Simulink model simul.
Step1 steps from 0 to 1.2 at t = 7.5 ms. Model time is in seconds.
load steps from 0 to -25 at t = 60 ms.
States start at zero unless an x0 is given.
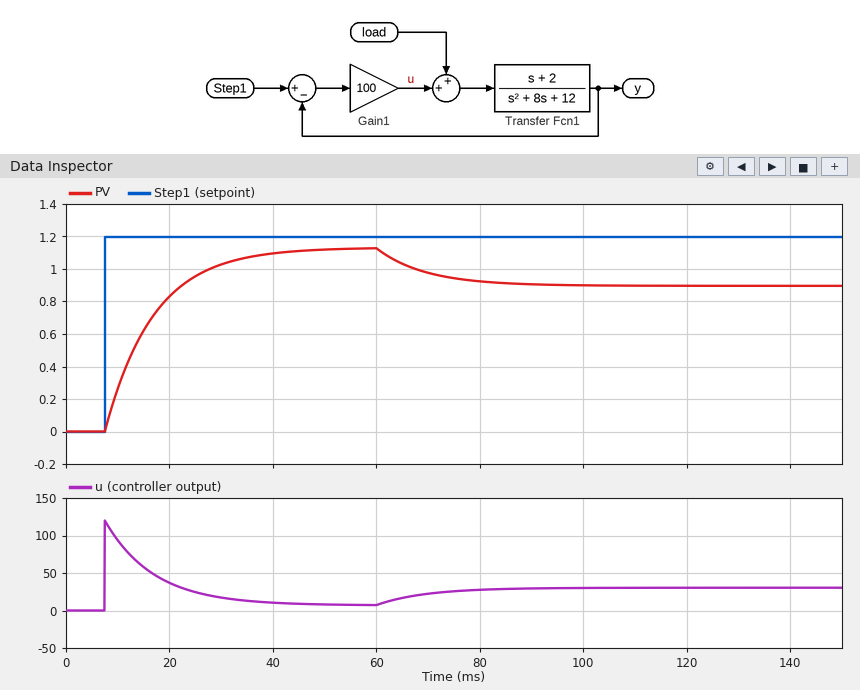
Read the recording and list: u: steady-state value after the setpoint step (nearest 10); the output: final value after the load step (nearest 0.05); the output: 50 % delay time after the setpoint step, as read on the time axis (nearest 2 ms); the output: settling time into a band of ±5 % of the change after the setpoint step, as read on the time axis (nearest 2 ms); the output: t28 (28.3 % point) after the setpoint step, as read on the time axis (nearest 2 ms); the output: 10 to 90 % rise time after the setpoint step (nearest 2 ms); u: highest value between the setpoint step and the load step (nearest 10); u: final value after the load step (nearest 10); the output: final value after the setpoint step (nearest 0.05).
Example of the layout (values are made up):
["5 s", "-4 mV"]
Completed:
["10", "0.90", "14 ms", "36 ms", "10 ms", "20 ms", "120", "30", "1.15"]
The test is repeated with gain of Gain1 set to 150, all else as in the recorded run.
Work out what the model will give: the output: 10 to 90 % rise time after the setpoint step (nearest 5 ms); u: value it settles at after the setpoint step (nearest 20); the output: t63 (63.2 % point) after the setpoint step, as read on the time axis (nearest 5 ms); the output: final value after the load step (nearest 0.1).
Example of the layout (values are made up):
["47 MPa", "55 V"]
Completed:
["15 ms", "0", "15 ms", "1.0"]
